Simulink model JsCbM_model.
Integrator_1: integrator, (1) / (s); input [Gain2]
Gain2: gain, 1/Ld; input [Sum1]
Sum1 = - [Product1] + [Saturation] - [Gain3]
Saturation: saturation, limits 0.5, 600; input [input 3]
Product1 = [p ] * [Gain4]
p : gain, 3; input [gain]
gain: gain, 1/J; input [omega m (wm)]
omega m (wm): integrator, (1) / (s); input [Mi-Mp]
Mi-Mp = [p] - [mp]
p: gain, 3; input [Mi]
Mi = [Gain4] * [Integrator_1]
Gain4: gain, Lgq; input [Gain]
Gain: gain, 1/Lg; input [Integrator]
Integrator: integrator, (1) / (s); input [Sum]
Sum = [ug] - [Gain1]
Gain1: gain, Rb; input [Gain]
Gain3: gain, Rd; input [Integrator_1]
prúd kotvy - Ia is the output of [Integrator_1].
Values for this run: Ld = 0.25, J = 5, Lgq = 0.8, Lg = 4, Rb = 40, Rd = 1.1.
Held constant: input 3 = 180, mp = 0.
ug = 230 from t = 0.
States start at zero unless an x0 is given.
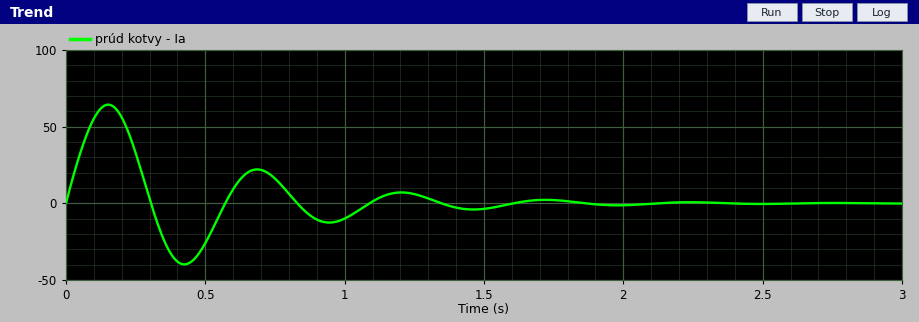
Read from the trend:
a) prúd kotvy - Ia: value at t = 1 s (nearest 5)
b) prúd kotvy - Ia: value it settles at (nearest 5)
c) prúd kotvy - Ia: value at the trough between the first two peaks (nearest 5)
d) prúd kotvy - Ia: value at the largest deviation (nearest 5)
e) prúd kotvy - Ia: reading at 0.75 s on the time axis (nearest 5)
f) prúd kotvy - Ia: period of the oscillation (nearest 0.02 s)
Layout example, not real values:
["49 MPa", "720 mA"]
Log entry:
["-10", "0", "-40", "65", "15", "0.54 s"]
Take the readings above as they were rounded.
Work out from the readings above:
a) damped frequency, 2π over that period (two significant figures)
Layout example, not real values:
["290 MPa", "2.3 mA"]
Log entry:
["12 rad/s"]
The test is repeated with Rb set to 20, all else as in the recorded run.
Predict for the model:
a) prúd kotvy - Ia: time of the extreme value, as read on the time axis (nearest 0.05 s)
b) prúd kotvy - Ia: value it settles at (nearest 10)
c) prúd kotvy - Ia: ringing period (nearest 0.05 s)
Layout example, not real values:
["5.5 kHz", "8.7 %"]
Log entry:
["0.15 s", "0", "0.35 s"]
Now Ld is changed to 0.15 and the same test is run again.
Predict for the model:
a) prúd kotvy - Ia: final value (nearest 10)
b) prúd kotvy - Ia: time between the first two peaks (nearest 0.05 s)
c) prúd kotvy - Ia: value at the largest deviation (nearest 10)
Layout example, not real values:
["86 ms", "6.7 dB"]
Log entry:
["0", "0.45 s", "80"]
